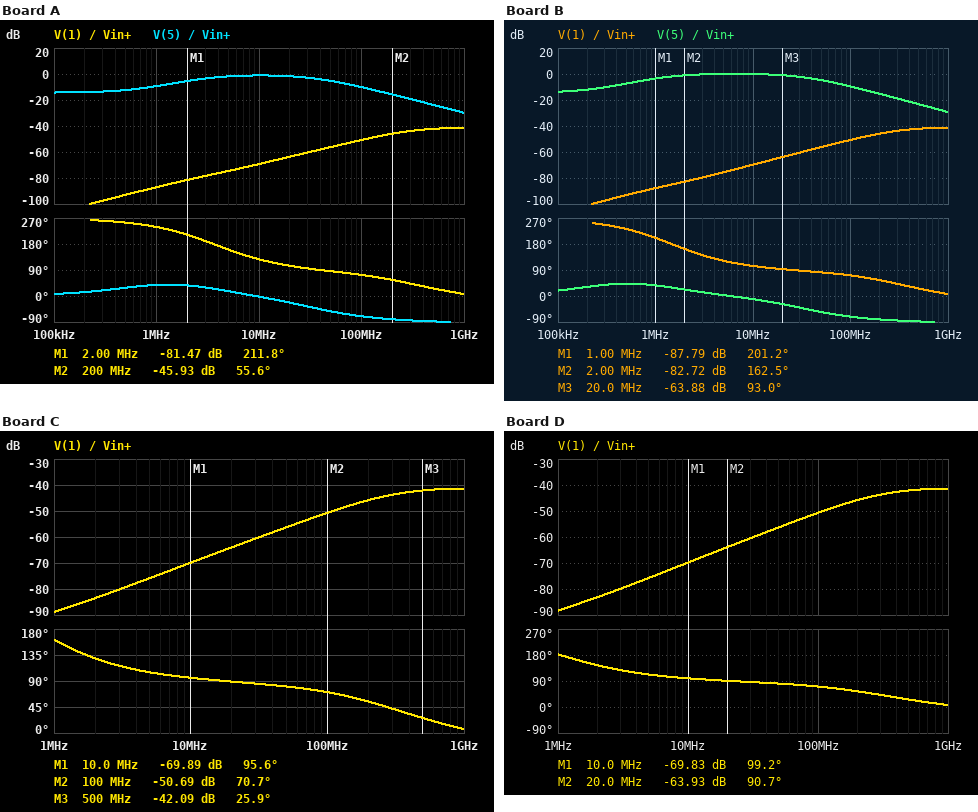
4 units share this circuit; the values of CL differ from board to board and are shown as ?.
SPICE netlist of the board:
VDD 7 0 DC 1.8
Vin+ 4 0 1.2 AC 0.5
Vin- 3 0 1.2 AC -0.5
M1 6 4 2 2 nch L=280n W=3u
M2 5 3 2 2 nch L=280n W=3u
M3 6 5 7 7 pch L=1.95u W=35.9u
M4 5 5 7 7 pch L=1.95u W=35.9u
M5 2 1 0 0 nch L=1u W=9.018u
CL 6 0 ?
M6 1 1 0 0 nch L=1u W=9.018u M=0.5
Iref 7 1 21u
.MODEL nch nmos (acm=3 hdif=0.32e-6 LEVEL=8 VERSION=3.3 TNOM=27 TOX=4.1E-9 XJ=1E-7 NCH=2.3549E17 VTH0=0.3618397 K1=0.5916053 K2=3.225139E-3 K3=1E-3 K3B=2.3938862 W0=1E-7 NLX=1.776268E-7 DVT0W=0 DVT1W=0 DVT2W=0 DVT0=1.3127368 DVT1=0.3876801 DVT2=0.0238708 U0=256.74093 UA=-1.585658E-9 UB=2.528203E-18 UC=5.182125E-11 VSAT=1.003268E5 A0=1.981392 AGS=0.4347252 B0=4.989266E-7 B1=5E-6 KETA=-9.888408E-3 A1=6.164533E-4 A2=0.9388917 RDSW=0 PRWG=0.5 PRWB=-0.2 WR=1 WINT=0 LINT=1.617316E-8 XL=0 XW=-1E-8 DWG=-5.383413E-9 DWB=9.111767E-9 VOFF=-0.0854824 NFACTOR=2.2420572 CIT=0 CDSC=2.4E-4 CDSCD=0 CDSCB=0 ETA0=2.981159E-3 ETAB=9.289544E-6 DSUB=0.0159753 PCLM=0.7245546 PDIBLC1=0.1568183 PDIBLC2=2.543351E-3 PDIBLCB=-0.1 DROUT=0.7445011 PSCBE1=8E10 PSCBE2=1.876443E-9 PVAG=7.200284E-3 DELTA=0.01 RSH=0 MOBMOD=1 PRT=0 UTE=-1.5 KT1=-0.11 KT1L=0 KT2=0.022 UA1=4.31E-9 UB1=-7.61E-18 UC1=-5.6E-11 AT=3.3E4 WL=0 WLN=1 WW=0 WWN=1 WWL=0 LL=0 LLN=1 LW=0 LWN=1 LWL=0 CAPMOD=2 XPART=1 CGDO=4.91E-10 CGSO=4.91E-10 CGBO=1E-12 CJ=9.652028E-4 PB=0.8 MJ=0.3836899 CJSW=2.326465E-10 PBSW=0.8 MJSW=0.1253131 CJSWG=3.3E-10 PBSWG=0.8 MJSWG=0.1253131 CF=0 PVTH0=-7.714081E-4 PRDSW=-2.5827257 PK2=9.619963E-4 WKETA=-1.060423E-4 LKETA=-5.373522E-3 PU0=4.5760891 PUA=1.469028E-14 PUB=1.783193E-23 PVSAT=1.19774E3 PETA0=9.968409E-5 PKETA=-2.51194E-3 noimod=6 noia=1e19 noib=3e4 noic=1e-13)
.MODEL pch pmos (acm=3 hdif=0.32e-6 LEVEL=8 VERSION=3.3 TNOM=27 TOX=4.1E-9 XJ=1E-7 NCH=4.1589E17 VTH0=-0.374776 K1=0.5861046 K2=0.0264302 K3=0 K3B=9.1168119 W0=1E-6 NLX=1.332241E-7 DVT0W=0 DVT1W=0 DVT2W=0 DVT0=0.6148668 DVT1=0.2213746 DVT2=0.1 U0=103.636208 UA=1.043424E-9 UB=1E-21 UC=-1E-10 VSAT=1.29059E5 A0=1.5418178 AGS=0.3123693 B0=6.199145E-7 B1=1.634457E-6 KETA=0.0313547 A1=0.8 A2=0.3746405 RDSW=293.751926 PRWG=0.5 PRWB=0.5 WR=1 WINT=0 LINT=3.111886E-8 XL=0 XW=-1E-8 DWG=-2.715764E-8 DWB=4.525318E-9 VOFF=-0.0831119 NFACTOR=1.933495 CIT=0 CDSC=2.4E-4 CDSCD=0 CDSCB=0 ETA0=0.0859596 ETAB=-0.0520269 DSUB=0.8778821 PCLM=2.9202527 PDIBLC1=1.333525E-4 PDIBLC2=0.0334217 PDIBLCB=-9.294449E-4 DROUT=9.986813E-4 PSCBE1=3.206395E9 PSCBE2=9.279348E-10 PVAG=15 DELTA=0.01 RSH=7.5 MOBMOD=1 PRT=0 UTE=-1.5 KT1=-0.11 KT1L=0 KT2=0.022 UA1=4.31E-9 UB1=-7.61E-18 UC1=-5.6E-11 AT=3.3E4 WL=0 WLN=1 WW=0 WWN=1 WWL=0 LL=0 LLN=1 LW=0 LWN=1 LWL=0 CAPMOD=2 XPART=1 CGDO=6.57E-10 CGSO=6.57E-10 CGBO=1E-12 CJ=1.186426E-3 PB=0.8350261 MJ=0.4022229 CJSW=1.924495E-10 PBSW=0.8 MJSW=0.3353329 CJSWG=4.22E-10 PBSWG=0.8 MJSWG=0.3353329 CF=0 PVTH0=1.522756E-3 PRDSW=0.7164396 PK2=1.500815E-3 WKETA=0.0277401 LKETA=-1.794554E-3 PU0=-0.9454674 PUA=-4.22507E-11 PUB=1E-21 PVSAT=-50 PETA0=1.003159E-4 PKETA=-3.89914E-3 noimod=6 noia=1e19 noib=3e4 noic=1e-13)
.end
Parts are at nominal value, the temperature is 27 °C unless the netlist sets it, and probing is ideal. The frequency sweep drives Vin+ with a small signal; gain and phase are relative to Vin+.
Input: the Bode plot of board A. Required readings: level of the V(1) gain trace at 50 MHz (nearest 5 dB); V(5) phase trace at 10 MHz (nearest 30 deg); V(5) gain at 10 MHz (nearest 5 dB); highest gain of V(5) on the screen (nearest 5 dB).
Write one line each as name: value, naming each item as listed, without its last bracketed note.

level of the V(1) gain trace at 50 MHz: -55 dB
V(5) phase trace at 10 MHz: 0 deg
V(5) gain at 10 MHz: 0 dB
highest gain of V(5) on the screen: 0 dB
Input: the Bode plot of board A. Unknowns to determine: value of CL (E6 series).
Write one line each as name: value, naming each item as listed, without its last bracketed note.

value of CL: 220 fF
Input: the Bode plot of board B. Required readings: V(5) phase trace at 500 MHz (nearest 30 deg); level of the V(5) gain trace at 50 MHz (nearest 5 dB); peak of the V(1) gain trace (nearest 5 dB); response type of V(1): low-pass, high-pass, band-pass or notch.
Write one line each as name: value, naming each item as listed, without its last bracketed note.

V(5) phase trace at 500 MHz: -90 deg
level of the V(5) gain trace at 50 MHz: -5 dB
peak of the V(1) gain trace: -40 dB
response type of V(1): low-pass, high-pass, band-pass or notch: high-pass
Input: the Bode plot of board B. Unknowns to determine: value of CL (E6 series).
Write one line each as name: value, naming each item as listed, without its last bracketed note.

value of CL: 680 fF
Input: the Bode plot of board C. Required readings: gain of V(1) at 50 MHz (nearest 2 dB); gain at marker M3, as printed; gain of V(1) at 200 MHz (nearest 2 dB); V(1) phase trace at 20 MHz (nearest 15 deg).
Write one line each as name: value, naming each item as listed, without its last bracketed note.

gain of V(1) at 50 MHz: -56 dB
gain at marker M3, as printed: -42.09 dB
gain of V(1) at 200 MHz: -46 dB
V(1) phase trace at 20 MHz: 90 deg
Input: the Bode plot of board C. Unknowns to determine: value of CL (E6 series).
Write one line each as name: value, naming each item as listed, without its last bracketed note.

value of CL: 1.5 pF
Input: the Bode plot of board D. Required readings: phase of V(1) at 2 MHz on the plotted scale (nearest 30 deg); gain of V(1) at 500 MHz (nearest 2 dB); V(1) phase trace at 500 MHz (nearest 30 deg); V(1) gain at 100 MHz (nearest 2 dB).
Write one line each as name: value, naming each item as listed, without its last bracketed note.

phase of V(1) at 2 MHz on the plotted scale: 150 deg
gain of V(1) at 500 MHz: -42 dB
V(1) phase trace at 500 MHz: 30 deg
V(1) gain at 100 MHz: -50 dB
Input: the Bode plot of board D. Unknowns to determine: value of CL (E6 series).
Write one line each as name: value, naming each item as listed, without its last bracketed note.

value of CL: 1 pF
